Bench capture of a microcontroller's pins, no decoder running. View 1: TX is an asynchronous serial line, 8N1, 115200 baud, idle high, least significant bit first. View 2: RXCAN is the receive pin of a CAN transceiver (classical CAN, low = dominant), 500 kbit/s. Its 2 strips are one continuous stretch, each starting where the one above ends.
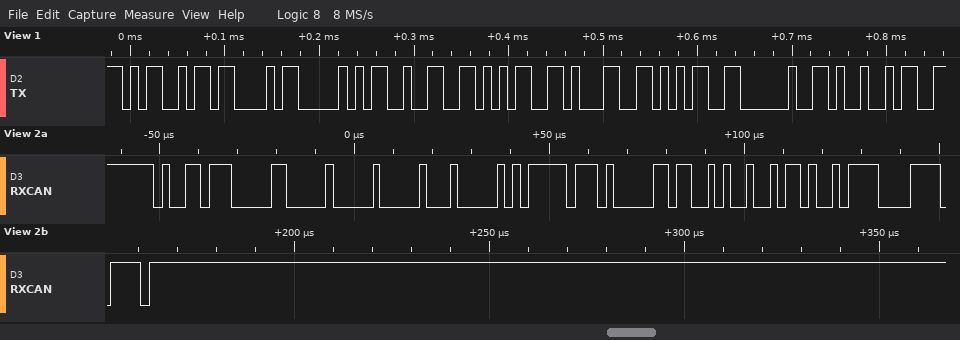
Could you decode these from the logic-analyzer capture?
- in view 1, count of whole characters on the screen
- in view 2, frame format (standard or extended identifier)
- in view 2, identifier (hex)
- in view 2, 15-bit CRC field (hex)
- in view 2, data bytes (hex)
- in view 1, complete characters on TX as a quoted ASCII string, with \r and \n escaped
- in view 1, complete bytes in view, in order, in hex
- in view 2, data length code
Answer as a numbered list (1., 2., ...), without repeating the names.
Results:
1. 9
2. standard
3. 0x4DC
4. 0x70F7
5. 00 01 02 FF 41 65 25 A5
6. "MCP2515 I"
7. 0x4D 0x43 0x50 0x32 0x35 0x31 0x35 0x20 0x49
8. 8
